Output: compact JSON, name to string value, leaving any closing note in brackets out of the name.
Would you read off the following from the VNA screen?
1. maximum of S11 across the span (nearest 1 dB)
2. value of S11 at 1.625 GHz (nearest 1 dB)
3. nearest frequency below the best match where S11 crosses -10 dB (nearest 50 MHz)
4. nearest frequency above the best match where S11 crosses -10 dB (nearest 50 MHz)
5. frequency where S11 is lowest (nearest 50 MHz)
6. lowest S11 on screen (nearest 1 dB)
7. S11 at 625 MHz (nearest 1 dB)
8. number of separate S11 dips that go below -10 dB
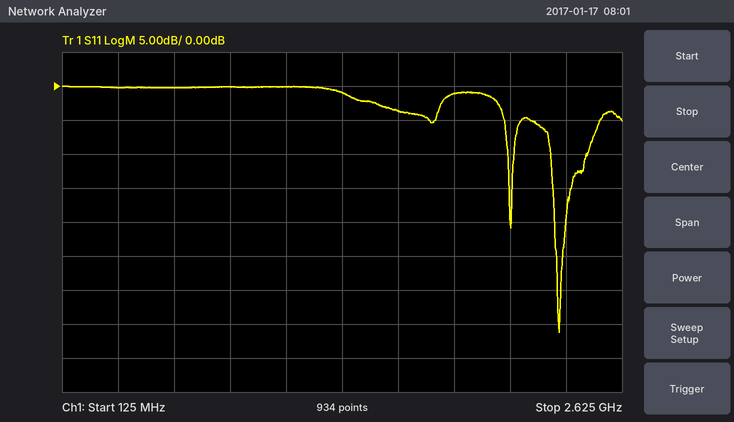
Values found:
{"maximum of S11 across the span": "0 dB", "value of S11 at 1.625 GHz": "-4 dB", "nearest frequency below the best match where S11 crosses -10 dB": "2.30 GHz", "nearest frequency above the best match where S11 crosses -10 dB": "2.45 GHz", "frequency where S11 is lowest": "2.35 GHz", "lowest S11 on screen": "-36 dB", "S11 at 625 MHz": "0 dB", "number of separate S11 dips that go below -10 dB": "2"}
